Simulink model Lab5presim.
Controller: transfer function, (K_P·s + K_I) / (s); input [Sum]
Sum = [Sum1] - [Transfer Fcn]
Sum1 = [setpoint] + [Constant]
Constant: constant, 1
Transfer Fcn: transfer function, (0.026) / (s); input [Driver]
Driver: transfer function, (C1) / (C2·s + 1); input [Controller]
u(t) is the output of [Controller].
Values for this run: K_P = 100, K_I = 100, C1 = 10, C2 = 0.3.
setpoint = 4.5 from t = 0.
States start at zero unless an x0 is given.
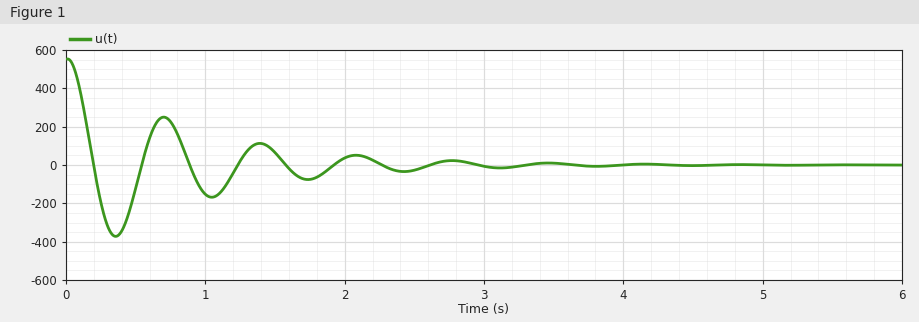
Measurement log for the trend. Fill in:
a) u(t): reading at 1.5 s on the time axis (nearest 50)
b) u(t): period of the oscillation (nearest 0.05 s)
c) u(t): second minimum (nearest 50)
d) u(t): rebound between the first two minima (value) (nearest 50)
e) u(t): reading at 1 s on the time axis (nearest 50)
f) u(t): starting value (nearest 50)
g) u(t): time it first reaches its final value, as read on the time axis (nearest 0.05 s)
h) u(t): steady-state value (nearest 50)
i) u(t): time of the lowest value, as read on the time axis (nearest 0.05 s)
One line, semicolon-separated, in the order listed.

50; 0.70 s; -150; 250; -150; 550; 0.20 s; 0; 0.35 s
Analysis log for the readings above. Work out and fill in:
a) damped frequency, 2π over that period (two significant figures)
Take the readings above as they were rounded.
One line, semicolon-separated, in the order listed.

9.0 rad/s
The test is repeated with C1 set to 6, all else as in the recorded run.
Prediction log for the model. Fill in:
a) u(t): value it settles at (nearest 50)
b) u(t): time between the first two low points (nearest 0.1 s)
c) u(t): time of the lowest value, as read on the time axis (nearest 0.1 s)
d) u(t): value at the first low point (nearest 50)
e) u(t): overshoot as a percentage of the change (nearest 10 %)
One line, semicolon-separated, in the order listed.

0; 0.9 s; 0.5 s; -350; 60 %
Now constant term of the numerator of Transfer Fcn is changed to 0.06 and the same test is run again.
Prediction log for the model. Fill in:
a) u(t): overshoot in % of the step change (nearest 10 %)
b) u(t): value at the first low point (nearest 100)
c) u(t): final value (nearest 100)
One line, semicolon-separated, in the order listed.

80 %; -400; 0
